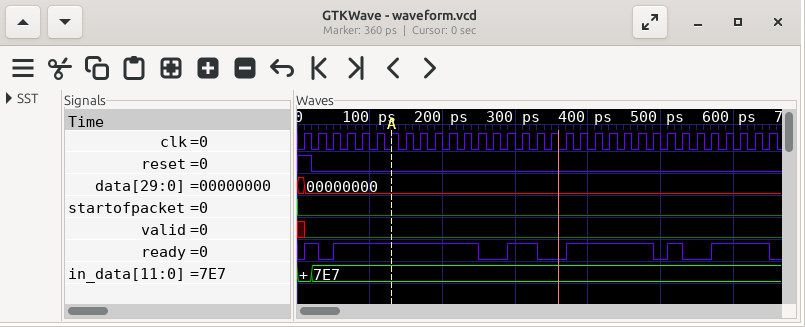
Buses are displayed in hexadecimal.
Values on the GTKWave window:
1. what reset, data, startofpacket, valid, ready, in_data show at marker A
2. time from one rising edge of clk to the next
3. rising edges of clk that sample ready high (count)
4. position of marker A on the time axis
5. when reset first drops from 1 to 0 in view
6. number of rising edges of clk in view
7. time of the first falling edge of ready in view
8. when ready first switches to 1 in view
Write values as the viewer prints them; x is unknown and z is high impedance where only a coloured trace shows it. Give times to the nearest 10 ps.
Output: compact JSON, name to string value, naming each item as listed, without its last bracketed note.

{"what reset, data, startofpacket, valid, ready, in_data show at marker A": "reset=0, data=00000000, startofpacket=0, valid=0, ready=1, in_data=7E7", "time from one rising edge of clk to the next": "20 ps", "rising edges of clk that sample ready high": "24", "position of marker A on the time axis": "130 ps", "when reset first drops from 1 to 0 in view": "20 ps", "number of rising edges of clk in view": "33", "time of the first falling edge of ready in view": "30 ps", "when ready first switches to 1 in view": "10 ps"}
